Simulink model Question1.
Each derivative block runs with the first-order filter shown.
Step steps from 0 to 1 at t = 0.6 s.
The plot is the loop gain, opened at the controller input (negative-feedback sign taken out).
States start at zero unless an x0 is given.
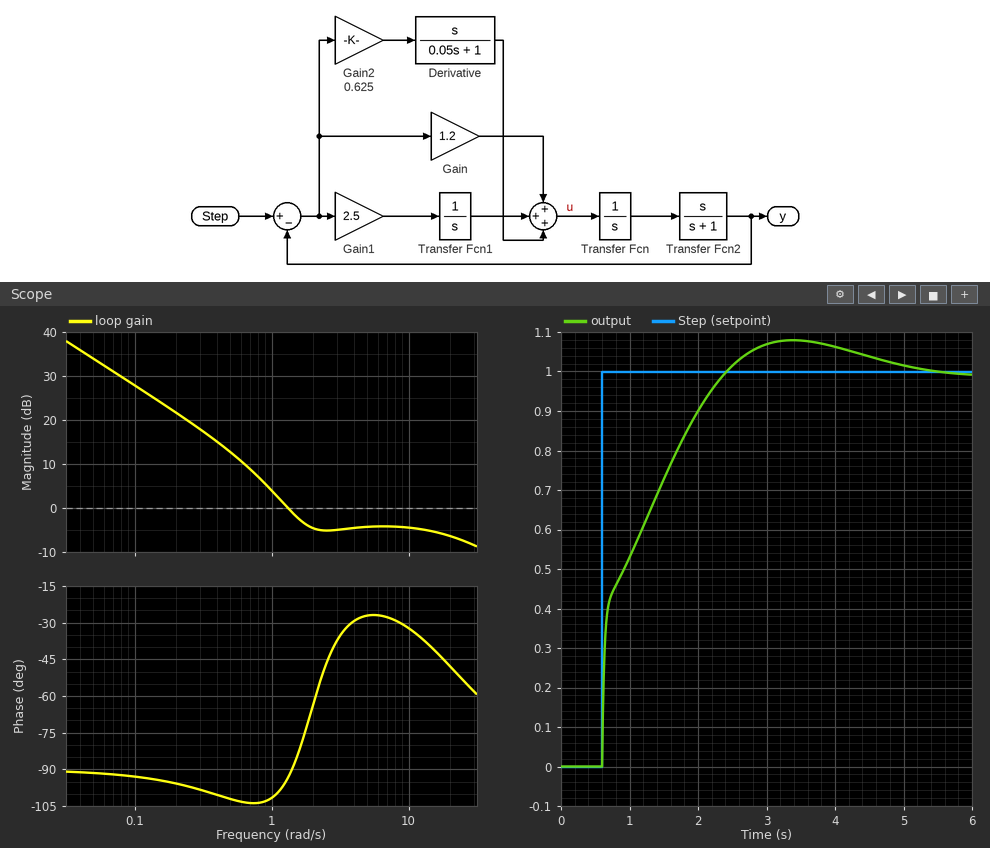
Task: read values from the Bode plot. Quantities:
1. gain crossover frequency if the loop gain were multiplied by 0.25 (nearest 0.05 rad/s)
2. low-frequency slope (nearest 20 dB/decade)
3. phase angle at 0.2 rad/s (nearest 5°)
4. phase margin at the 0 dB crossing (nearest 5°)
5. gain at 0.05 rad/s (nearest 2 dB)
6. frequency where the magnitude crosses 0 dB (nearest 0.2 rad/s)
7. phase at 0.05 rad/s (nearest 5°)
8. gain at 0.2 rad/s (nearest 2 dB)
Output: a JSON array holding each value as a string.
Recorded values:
["0.55 rad/s", "-20 dB/decade", "-95°", "85°", "34 dB", "1.4 rad/s", "-90°", "22 dB"]
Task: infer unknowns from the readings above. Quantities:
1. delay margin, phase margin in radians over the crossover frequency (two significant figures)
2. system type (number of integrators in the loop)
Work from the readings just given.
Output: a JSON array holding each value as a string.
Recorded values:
["1.1 s", "1"]
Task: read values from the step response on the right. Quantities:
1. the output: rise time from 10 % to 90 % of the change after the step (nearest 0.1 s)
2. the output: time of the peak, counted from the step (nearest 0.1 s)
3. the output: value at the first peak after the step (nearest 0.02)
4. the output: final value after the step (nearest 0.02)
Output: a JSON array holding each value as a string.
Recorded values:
["1.4 s", "2.8 s", "1.08", "1.00"]
